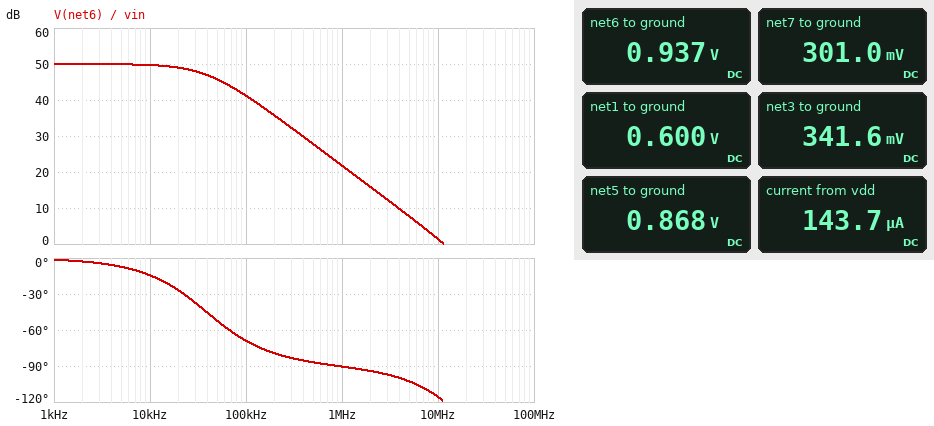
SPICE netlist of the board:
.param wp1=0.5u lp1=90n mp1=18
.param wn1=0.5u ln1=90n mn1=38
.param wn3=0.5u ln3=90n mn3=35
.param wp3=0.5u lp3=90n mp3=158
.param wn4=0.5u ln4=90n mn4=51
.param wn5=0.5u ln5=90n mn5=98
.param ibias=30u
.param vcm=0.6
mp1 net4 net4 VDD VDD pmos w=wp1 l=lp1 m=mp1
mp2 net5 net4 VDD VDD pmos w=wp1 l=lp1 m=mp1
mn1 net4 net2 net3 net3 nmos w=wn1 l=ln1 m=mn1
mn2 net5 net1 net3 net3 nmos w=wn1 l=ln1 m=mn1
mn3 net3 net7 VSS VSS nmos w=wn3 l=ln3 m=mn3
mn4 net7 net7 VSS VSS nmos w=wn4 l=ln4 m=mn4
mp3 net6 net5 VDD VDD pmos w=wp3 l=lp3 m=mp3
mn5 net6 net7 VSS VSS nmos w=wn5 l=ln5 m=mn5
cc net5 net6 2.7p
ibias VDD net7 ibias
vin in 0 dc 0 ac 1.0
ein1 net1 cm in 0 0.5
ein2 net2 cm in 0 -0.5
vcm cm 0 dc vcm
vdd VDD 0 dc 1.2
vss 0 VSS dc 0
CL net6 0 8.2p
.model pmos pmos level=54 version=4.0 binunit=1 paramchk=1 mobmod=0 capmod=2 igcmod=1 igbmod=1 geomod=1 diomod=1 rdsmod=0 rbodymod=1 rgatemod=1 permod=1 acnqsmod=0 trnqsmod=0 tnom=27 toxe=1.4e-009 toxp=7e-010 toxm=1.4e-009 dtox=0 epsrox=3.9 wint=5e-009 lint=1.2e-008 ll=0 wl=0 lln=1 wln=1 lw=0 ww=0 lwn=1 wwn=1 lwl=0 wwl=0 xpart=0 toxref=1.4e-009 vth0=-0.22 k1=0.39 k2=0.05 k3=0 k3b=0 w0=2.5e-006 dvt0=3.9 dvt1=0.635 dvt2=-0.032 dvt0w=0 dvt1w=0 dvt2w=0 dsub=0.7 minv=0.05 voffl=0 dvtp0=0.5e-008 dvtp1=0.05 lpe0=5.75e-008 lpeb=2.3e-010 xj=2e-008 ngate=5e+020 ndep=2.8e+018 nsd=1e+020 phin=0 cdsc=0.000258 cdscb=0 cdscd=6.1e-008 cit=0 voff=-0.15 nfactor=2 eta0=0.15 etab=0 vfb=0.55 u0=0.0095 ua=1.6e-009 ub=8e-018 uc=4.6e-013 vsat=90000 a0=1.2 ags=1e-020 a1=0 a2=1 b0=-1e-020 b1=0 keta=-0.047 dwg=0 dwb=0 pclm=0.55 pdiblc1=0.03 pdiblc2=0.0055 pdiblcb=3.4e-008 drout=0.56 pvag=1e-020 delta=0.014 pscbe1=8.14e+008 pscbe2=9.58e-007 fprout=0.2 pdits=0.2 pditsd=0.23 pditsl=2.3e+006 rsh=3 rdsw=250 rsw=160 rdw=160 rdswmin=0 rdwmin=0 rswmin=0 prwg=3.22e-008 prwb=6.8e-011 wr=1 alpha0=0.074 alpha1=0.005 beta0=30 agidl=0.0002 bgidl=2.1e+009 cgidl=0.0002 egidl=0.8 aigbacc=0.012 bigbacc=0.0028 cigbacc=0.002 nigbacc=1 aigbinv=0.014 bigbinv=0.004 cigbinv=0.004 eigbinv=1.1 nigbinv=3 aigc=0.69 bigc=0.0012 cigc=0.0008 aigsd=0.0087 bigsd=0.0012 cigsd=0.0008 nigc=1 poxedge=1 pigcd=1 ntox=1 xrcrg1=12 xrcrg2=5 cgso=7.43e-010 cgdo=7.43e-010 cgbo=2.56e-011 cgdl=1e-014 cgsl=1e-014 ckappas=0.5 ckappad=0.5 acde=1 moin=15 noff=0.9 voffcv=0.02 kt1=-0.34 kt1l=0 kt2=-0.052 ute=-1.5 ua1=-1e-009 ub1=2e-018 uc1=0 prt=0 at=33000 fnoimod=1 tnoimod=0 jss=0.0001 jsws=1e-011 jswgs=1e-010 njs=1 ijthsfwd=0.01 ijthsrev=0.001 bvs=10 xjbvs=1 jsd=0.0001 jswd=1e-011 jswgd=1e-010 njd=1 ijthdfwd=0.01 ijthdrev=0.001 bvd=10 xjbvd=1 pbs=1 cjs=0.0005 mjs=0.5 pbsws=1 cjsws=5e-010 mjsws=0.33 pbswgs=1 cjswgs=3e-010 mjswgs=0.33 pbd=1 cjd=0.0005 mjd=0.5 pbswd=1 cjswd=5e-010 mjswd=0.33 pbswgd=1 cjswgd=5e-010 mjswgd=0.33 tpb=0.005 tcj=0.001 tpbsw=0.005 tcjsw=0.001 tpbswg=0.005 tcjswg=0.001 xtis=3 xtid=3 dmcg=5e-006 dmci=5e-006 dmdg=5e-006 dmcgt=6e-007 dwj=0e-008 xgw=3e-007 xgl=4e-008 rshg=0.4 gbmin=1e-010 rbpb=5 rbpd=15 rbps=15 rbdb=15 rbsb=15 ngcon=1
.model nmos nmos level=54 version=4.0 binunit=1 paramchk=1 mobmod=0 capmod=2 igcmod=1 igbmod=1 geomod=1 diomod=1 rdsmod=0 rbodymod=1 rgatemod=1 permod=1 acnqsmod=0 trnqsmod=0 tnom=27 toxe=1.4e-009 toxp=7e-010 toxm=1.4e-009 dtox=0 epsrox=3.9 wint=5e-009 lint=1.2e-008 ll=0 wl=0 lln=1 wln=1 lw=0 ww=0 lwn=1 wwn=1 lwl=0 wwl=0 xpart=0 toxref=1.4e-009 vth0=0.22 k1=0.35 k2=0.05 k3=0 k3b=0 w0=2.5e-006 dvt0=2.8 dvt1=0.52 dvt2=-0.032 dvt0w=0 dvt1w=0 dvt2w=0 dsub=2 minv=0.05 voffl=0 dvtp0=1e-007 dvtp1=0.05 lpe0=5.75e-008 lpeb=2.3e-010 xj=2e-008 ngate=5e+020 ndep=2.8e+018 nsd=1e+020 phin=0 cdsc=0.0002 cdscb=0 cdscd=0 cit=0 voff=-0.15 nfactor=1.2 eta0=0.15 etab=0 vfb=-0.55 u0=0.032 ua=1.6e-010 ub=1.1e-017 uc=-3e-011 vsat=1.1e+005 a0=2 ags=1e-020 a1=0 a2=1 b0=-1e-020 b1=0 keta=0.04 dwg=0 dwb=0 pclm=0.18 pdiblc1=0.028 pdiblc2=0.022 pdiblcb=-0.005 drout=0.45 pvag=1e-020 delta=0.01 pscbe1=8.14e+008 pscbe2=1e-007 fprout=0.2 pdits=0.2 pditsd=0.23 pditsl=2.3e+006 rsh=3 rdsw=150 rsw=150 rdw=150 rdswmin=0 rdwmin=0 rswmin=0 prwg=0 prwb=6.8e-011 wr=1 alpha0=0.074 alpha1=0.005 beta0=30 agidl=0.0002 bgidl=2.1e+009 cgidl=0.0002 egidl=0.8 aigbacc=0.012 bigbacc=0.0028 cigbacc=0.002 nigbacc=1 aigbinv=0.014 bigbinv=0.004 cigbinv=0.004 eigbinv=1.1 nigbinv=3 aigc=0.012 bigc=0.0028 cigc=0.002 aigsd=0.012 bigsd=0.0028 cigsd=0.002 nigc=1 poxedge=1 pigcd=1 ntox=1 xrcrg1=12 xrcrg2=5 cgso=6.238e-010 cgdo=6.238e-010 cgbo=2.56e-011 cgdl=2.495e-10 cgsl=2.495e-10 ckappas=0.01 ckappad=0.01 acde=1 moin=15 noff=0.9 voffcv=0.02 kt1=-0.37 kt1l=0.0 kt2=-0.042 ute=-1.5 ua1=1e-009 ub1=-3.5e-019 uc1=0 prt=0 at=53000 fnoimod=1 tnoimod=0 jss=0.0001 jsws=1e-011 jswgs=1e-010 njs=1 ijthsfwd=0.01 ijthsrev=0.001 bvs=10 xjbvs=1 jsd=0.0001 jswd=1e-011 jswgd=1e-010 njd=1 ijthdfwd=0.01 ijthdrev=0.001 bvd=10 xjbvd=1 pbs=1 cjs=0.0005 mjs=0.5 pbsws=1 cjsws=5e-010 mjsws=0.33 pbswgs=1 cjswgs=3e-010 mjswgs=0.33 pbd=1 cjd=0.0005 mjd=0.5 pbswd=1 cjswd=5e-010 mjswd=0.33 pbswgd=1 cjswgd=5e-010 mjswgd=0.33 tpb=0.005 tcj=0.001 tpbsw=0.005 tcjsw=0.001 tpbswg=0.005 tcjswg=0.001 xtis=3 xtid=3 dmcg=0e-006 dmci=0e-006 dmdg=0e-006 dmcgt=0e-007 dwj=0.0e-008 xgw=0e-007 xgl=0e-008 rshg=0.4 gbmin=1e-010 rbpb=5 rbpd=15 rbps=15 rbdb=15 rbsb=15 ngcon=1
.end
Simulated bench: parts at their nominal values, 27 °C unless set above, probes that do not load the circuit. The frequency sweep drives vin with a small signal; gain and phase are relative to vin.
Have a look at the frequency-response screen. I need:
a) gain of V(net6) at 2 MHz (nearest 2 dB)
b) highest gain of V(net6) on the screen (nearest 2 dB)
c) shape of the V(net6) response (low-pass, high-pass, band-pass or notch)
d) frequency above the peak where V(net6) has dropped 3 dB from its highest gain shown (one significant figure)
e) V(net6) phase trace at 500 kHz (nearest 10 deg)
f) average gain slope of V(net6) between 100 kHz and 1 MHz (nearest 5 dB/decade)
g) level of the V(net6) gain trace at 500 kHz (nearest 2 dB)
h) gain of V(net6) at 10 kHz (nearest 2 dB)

16 dB
50 dB
low-pass
40 kHz
-90 deg
-20 dB/decade
28 dB
50 dB
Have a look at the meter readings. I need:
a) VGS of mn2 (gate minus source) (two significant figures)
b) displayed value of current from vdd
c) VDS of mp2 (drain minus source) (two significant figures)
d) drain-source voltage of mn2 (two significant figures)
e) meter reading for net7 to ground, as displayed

260 mV
143.7 µA
-330 mV
530 mV
301.0 mV
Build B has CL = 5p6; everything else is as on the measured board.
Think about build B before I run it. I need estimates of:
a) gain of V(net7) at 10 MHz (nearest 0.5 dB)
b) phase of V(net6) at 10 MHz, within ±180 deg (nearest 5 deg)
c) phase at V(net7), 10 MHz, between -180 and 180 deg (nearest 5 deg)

-35.0 dB
-110 deg
-100 deg
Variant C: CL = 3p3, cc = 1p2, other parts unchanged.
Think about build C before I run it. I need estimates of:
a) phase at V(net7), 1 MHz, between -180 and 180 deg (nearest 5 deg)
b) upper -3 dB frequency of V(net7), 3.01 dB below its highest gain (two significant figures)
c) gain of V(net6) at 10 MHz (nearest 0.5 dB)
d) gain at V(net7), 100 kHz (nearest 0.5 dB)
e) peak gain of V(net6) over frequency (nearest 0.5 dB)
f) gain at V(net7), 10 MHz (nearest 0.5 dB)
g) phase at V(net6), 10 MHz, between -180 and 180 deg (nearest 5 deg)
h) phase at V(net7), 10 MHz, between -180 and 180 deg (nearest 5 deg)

-85 deg
85 kHz
8.5 dB
9.0 dB
50.0 dB
-28.5 dB
-105 deg
-90 deg
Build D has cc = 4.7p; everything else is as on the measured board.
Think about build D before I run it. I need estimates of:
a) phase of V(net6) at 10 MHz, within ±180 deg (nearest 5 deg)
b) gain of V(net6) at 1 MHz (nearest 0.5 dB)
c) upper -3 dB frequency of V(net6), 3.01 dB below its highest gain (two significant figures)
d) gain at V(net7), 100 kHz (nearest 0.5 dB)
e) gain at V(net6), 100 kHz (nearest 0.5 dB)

-120 deg
17.0 dB
23 kHz
0 dB
37.0 dB
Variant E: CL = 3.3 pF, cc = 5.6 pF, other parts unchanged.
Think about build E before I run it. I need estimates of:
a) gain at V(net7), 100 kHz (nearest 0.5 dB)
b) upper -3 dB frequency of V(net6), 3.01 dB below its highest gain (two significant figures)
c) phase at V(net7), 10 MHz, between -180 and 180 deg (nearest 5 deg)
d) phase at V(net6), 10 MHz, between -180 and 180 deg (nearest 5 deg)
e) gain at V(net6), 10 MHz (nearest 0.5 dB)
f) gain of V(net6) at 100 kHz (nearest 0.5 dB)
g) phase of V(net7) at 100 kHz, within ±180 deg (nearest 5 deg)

-1.5 dB
19 kHz
-100 deg
-110 deg
-4.0 dB
35.5 dB
-80 deg
